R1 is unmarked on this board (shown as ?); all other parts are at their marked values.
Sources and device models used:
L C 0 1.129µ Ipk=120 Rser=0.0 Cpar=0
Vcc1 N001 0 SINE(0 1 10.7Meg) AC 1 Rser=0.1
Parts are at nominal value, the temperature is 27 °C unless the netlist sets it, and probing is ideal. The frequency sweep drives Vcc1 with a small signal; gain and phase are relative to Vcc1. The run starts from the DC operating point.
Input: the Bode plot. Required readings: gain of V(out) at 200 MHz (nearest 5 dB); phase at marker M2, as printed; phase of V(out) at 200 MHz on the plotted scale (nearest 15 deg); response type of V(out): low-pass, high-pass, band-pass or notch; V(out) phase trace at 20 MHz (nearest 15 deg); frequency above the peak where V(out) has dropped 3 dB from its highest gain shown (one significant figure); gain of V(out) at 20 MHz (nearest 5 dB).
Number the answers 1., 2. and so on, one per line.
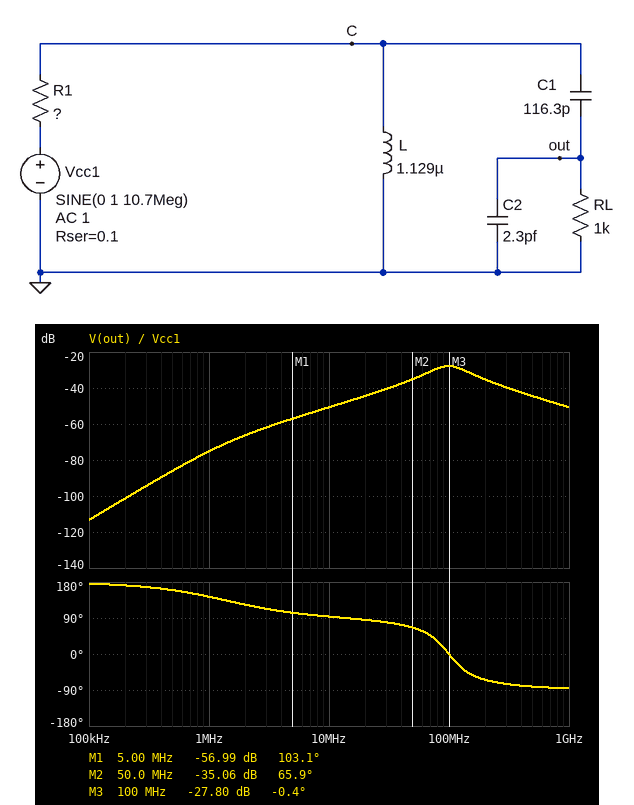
1. -35 dB
2. 65.9 deg
3. -60 deg
4. band-pass
5. 90 deg
6. 100 MHz
7. -45 dB
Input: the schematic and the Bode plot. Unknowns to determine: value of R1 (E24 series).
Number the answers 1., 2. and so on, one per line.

1. 24 kΩ
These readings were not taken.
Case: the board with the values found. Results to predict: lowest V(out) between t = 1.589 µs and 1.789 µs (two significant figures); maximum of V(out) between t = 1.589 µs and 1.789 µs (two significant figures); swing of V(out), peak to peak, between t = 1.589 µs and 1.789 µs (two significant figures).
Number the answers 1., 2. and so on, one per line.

1. -3.1 mV
2. 3.1 mV
3. 6.3 mV
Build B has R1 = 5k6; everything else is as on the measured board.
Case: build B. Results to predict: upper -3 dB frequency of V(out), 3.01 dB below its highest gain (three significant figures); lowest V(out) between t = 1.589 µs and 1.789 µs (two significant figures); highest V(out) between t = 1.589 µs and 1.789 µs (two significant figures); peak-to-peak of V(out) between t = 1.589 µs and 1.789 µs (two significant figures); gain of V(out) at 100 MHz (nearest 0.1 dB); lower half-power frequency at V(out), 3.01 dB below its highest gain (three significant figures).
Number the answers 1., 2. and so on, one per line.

1. 147 MHz
2. -13 mV
3. 13 mV
4. 27 mV
5. -16.3 dB
6. 66.9 MHz
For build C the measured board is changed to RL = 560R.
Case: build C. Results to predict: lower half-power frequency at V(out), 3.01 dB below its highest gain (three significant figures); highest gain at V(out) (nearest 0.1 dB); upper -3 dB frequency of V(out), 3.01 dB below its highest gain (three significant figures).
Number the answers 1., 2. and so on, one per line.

1. 54.2 MHz
2. -32.7 dB
3. 178 MHz
